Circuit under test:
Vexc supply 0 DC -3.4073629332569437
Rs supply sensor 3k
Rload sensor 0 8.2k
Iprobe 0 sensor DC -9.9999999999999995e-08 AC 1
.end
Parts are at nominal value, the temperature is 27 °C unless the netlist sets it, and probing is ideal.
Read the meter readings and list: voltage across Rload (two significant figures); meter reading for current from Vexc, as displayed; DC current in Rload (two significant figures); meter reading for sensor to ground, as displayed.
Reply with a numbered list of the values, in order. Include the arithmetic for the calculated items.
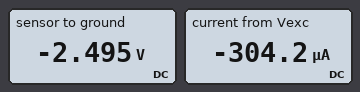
1. 0 V - (-2.495 V) = 2.5 V
2. -304.2 µA
3. (0 V - (-2.495 V)) / 8.2 kΩ = 300 µA
4. -2.495 V
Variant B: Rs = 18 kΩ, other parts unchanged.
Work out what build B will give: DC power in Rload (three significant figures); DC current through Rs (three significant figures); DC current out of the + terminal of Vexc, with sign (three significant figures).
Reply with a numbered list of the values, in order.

1. 139 µW
2. 130 µA
3. -130 µA
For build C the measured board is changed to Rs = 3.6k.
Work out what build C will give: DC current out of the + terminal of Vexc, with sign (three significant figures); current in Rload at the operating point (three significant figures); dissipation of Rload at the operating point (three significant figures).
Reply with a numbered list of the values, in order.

1. -289 µA
2. 289 µA
3. 684 µW
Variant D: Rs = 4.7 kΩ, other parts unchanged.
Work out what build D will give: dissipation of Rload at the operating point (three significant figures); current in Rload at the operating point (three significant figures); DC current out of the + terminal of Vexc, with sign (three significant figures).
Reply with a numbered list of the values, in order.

1. 572 µW
2. 264 µA
3. -264 µA
